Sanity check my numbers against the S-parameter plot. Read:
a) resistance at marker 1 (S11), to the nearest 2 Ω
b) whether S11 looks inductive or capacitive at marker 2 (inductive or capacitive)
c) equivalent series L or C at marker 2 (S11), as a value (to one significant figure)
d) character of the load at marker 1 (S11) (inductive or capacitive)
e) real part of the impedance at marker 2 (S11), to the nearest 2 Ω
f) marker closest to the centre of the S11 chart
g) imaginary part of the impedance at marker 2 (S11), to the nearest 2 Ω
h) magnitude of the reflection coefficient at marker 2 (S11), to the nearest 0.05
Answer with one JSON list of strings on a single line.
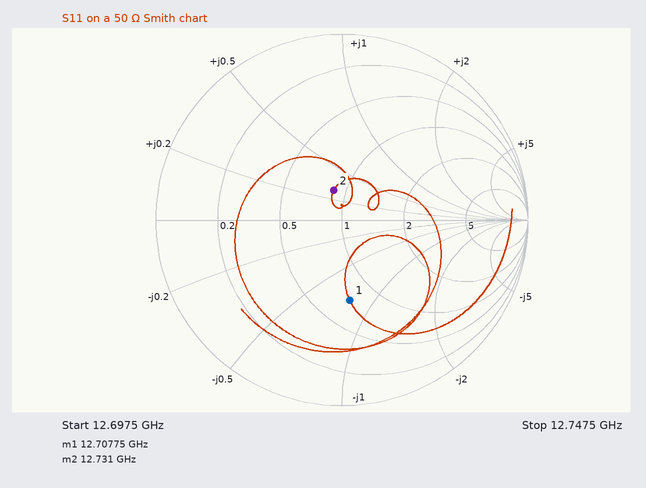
["36 Ω", "inductive", "200 pH", "capacitive", "44 Ω", "marker 2", "+14 Ω", "0.15"]
